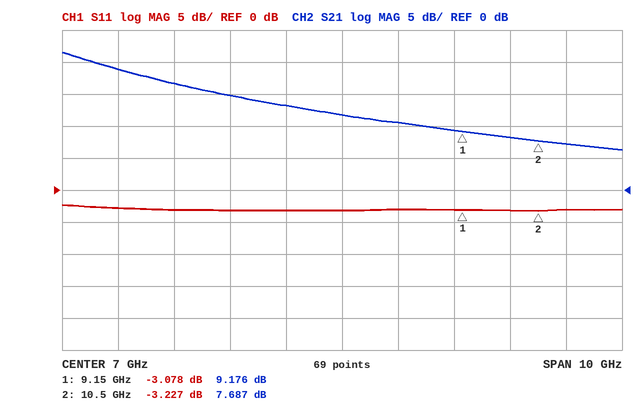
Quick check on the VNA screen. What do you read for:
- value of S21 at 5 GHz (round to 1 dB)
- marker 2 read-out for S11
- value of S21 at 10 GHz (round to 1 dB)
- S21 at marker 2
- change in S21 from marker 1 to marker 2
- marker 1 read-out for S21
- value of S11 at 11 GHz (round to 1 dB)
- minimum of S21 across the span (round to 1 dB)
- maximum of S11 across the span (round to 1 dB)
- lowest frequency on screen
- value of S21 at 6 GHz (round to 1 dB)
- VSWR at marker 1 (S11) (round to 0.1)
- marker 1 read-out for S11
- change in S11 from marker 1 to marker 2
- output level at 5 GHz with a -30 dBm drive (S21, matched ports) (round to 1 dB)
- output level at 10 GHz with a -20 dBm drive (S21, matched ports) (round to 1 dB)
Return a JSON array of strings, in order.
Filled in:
["15 dB", "-3.227 dB", "8 dB", "7.687 dB", "-1.489 dB", "9.176 dB", "-3 dB", "6 dB", "-2 dB", "2 GHz", "13 dB", "5.7", "-3.078 dB", "-0.149 dB", "-15 dBm", "-12 dBm"]
